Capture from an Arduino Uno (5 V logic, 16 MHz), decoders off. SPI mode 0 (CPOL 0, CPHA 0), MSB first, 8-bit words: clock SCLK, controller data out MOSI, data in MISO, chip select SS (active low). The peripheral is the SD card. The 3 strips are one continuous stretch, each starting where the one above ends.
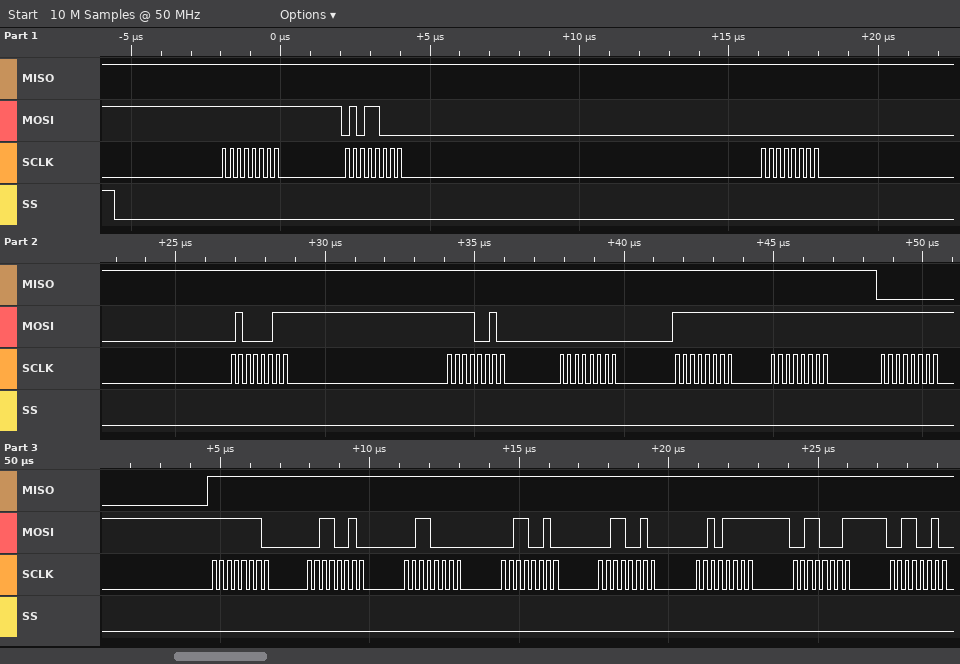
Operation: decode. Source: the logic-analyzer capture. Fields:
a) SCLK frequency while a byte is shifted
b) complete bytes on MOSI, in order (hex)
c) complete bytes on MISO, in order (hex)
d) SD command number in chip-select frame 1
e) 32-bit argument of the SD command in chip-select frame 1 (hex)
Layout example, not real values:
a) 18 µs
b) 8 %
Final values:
a) 4 MHz
b) FF 58 00 43 F2 00 FF FF FF FE 32 30 32 32 2F 31 32
c) FF FF FF FF FF FF FF FF 00 FF FF FF FF FF FF FF FF
d) CMD24
e) 0x0043F200
